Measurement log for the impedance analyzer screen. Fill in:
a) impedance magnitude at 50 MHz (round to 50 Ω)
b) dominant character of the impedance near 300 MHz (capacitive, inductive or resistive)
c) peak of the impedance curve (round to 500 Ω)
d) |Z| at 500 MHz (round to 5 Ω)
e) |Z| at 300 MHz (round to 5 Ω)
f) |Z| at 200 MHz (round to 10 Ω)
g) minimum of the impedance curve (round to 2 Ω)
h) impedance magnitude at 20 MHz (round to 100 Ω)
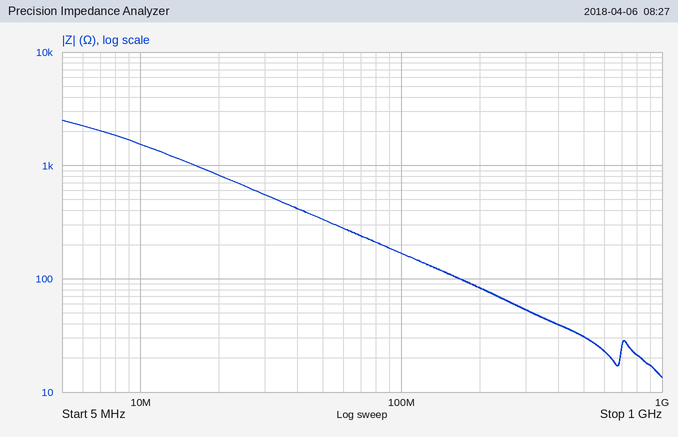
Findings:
350 Ω
capacitive
2.5 kΩ
30 Ω
55 Ω
80 Ω
14 Ω
800 Ω
